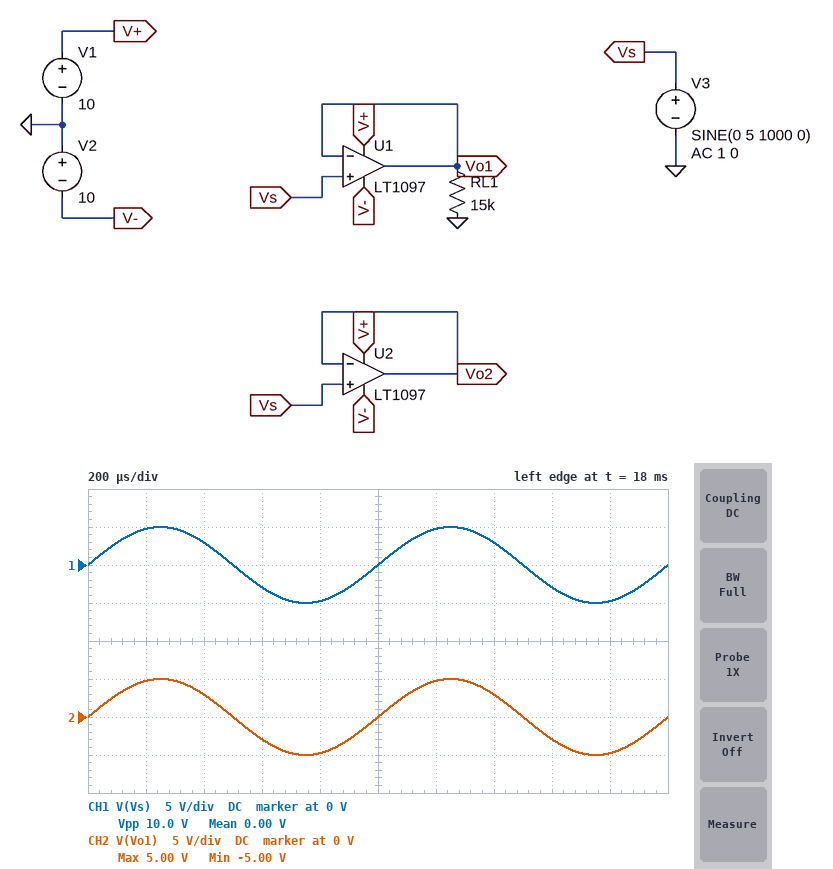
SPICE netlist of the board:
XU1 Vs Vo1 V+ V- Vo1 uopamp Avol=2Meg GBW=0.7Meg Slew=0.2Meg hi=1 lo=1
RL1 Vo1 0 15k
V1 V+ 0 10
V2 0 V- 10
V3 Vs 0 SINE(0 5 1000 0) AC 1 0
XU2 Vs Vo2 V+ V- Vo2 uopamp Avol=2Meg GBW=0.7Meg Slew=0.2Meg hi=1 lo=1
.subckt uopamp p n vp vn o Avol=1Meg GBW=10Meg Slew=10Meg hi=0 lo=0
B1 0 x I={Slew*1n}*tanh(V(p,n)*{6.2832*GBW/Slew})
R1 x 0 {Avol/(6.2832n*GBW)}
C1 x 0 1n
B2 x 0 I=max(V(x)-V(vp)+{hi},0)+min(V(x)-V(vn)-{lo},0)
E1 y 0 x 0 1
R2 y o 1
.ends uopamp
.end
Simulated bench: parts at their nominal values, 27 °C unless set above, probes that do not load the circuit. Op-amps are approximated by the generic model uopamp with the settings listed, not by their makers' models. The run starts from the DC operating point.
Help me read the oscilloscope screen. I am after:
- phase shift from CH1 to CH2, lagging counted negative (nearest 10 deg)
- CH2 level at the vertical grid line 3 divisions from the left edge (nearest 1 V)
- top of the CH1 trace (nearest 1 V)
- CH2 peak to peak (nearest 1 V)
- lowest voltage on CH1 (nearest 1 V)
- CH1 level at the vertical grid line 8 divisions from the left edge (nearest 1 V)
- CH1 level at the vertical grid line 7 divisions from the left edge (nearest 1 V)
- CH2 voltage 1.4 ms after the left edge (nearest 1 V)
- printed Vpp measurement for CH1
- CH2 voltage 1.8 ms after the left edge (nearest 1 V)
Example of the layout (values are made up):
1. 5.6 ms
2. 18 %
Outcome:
1. 0 deg
2. -3 V
3. 5 V
4. 10 V
5. -5 V
6. -3 V
7. 3 V
8. 3 V
9. 10.0 V
10. -5 V
